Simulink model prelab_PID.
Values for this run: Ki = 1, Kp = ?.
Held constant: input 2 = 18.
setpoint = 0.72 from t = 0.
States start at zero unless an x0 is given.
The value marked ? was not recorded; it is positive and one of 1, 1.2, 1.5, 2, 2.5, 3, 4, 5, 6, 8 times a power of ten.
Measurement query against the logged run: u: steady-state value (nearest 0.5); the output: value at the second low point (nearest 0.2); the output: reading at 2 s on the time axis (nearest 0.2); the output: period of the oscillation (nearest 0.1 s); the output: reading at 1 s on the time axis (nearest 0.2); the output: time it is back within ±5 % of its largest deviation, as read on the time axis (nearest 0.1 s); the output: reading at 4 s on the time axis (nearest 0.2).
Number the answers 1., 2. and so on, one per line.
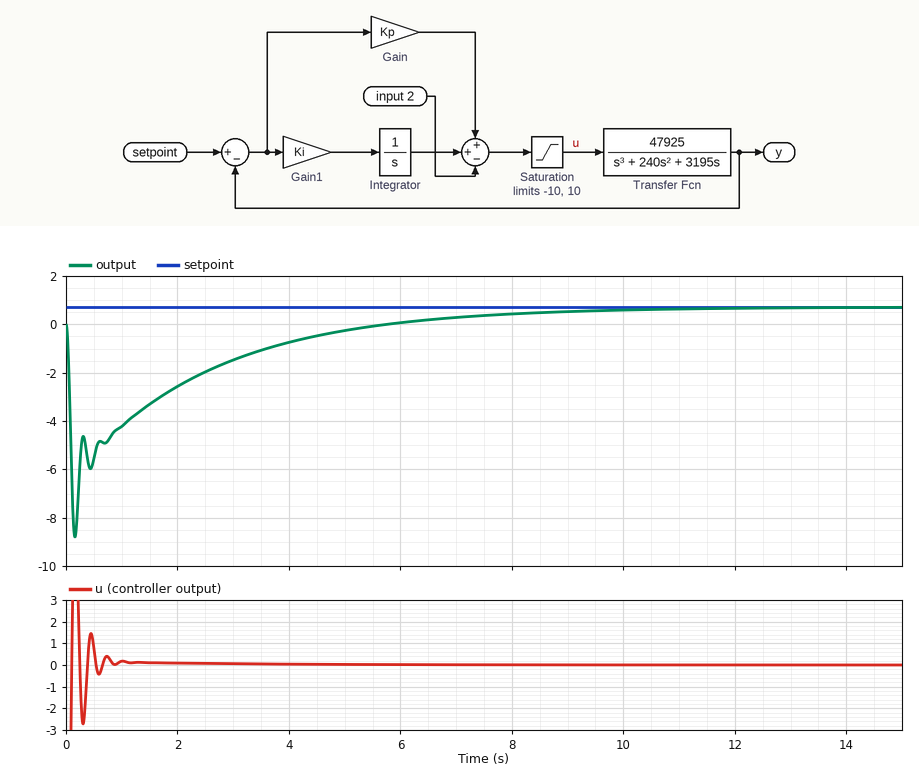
1. 0.0
2. -6.0
3. -2.6
4. 0.3 s
5. -4.2
6. 7.0 s
7. -0.8
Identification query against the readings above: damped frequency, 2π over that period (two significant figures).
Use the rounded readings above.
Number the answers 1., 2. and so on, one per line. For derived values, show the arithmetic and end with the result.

1. 2π / 0.3 = 21 rad/s
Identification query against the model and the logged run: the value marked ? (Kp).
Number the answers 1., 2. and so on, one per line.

1. 2.5
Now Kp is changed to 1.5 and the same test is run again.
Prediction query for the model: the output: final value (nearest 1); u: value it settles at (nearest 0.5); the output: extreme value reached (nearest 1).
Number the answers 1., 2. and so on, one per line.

1. 1
2. 0.0
3. -14
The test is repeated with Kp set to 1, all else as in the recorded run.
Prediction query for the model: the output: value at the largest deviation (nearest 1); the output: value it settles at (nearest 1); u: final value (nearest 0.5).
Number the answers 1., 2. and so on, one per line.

1. -19
2. 1
3. 0.0
